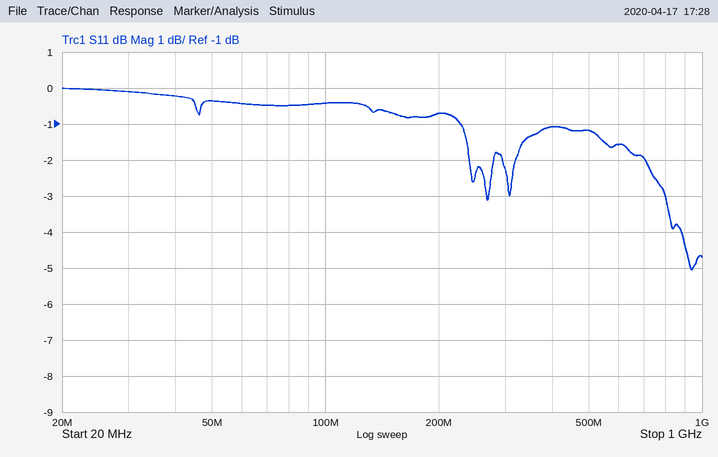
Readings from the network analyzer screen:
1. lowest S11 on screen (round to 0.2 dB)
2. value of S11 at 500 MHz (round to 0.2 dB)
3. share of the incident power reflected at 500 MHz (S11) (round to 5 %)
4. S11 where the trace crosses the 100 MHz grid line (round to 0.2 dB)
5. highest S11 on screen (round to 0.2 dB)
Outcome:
-5.0 dB
-1.2 dB
75 %
-0.4 dB
0.0 dB
